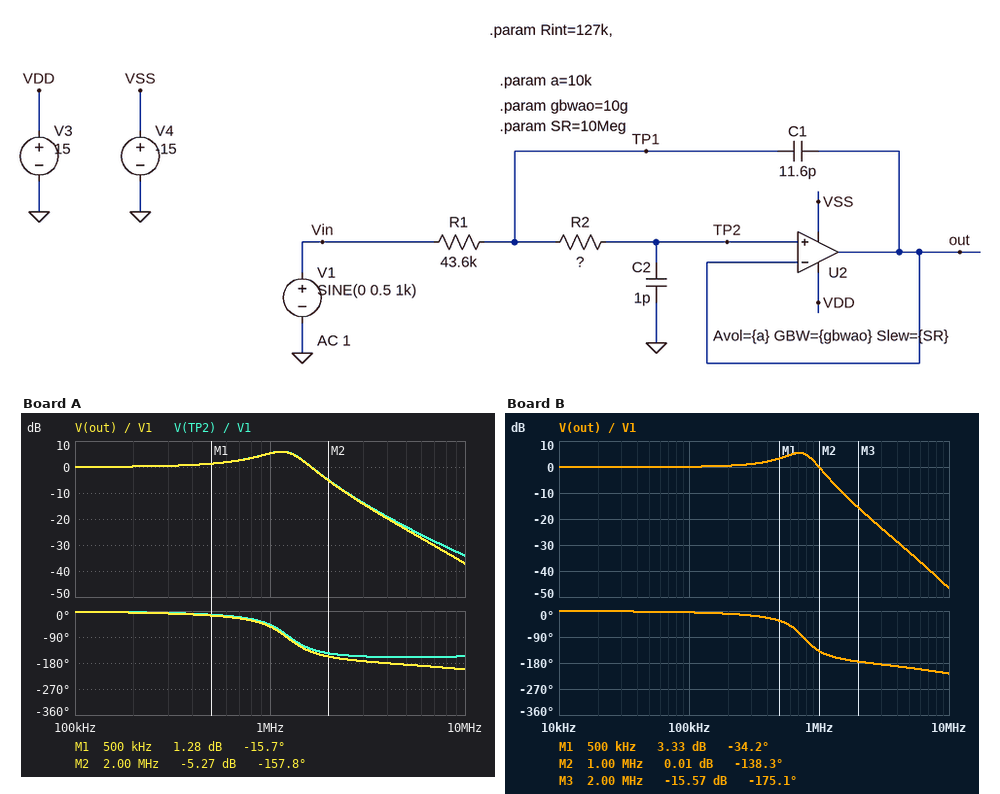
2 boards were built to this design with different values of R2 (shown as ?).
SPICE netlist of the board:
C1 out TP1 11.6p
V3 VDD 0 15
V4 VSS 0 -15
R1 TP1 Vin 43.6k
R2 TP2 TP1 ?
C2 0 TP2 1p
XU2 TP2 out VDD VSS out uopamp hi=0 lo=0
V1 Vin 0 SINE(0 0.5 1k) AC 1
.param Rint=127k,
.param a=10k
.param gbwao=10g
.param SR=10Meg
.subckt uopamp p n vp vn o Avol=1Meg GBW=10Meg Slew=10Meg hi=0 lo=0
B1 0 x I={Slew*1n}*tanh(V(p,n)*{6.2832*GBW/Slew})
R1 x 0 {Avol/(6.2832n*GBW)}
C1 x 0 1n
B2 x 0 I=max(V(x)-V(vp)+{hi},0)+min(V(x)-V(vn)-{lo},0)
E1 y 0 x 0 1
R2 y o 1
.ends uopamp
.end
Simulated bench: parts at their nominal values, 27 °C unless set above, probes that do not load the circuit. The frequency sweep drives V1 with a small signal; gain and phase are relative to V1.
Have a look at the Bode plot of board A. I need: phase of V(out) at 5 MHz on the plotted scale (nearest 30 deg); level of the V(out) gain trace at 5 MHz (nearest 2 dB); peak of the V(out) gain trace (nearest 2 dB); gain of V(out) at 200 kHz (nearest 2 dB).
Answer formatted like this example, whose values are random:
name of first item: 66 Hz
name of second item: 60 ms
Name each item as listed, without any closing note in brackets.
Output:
phase of V(out) at 5 MHz on the plotted scale: -180 deg
level of the V(out) gain trace at 5 MHz: -24 dB
peak of the V(out) gain trace: 6 dB
gain of V(out) at 200 kHz: 0 dB
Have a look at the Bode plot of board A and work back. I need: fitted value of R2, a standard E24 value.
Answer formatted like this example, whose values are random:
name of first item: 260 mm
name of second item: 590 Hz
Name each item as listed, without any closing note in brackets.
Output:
fitted value of R2, a standard E24 value: 16 kΩ
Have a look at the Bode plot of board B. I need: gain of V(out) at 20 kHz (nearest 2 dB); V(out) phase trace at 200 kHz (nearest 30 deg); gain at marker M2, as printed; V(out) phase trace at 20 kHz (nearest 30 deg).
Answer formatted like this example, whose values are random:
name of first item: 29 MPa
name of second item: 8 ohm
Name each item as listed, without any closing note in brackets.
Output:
gain of V(out) at 20 kHz: 0 dB
V(out) phase trace at 200 kHz: 0 deg
gain at marker M2, as printed: 0.01 dB
V(out) phase trace at 20 kHz: 0 deg
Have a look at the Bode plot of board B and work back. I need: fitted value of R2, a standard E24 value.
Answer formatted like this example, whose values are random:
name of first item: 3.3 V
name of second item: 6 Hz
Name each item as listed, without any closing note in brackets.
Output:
fitted value of R2, a standard E24 value: 68 kΩ
